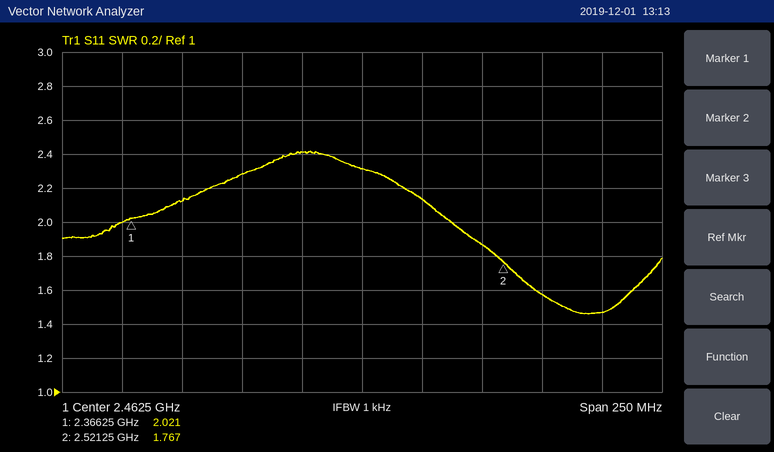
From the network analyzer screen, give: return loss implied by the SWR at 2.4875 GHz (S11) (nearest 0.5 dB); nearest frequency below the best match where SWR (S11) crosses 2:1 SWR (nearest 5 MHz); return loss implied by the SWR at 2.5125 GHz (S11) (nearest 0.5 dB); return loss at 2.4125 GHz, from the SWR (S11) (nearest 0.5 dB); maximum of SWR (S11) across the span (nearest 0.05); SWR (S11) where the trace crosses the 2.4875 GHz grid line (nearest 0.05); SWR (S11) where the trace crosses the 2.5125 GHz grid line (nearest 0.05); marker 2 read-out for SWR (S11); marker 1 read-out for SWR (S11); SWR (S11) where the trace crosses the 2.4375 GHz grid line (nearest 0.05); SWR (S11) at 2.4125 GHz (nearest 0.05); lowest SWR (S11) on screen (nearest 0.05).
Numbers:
9.0 dB
2.500 GHz
10.5 dB
8.0 dB
2.40
2.15
1.85
1.767
2.021
2.40
2.30
1.45
